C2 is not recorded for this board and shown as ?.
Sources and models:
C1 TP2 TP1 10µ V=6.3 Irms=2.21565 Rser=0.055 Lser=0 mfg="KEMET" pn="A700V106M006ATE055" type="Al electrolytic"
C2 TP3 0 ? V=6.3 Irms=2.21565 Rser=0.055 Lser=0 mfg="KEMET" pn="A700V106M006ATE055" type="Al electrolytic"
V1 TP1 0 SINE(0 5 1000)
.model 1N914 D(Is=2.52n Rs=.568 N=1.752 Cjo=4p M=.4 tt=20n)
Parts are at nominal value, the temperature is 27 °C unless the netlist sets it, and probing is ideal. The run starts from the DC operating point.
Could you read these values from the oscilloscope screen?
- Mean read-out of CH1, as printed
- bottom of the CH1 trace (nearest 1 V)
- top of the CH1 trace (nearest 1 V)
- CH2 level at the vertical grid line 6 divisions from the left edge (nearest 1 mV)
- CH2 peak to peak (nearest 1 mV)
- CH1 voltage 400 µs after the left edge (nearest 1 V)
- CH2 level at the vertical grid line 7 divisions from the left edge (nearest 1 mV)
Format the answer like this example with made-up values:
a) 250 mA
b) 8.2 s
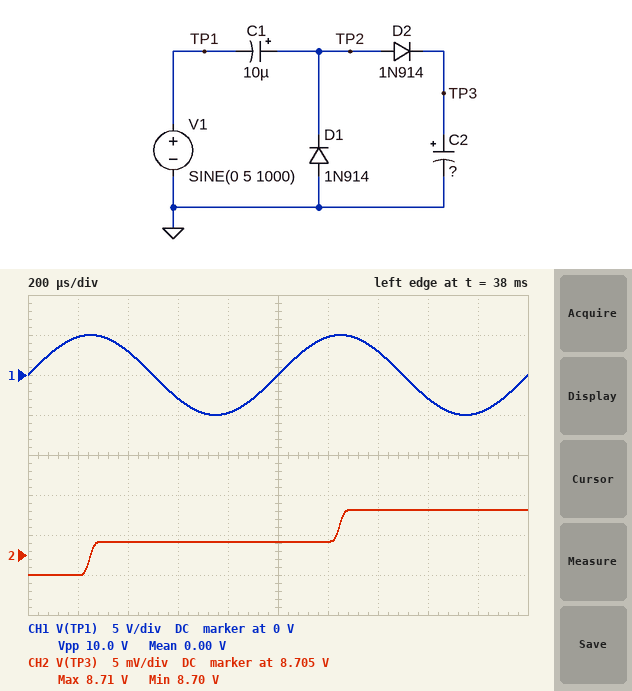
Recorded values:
a) 0.00 V
b) -5 V
c) 5 V
d) 8.707 V
e) 8 mV
f) 3 V
g) 8.711 V
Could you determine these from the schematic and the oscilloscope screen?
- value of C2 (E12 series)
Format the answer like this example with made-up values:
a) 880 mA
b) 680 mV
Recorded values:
a) 33 µF
